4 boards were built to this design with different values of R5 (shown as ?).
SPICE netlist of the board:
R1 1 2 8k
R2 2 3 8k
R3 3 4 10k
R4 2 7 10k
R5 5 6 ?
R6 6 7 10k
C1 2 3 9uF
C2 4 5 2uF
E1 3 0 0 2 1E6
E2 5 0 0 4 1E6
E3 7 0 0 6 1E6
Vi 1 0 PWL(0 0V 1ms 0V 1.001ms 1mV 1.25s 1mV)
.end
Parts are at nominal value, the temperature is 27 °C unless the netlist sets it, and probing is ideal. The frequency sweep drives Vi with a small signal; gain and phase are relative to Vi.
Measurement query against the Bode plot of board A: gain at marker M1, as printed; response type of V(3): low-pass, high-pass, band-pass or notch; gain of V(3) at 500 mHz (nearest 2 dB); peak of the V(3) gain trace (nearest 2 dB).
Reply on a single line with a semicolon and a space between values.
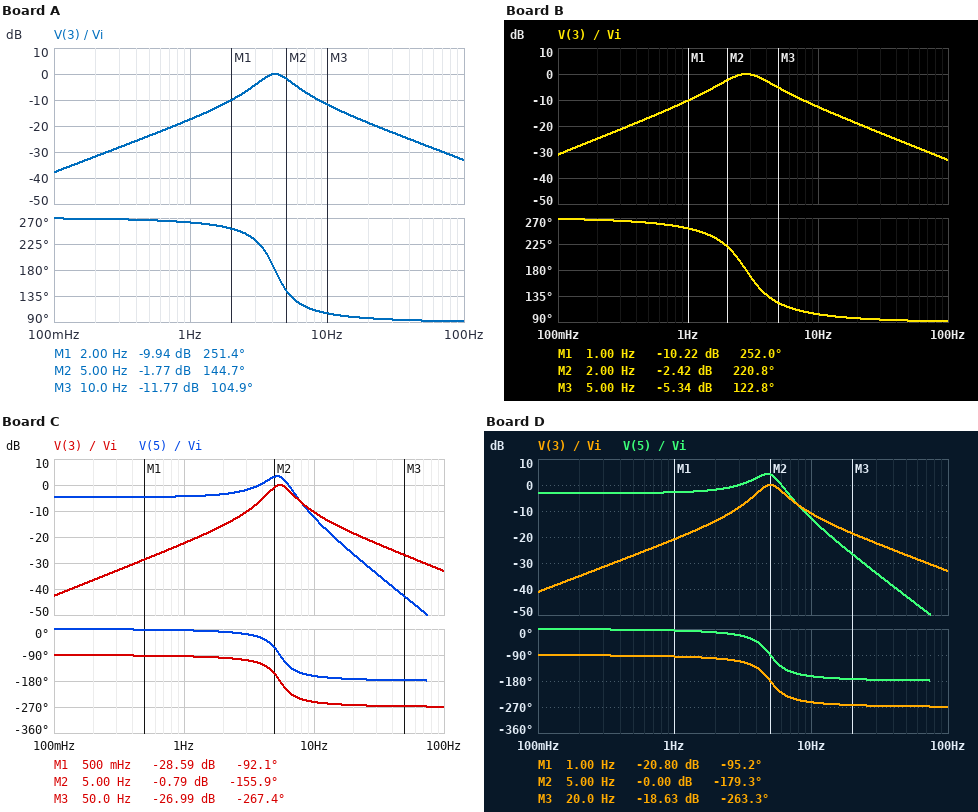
-9.94 dB; band-pass; -24 dB; 0 dB
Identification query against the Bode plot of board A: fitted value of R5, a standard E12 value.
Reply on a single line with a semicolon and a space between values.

8.2 kΩ
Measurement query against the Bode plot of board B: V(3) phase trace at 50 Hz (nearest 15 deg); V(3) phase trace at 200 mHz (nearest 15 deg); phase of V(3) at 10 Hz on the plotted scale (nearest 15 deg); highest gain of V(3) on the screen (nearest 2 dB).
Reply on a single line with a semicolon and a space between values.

90 deg; 270 deg; 105 deg; 0 dB
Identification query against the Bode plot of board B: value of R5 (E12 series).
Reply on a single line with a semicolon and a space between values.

18 kΩ
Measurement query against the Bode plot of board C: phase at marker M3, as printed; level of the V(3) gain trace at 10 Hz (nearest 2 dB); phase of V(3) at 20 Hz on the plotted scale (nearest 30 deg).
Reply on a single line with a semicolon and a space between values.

-267.4 deg; -10 dB; -270 deg
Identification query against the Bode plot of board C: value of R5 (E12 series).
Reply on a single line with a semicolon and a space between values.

4.7 kΩ
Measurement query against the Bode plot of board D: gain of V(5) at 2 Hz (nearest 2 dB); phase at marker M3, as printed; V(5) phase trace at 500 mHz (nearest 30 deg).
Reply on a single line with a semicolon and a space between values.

-2 dB; -263.3 deg; 0 deg
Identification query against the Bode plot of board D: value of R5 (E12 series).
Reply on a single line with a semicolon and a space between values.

5.6 kΩ
